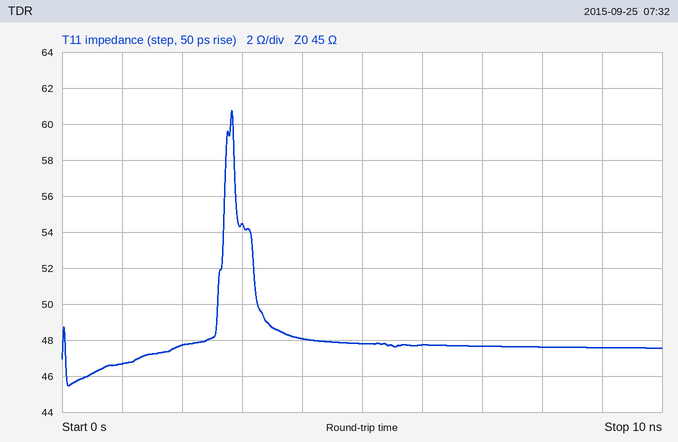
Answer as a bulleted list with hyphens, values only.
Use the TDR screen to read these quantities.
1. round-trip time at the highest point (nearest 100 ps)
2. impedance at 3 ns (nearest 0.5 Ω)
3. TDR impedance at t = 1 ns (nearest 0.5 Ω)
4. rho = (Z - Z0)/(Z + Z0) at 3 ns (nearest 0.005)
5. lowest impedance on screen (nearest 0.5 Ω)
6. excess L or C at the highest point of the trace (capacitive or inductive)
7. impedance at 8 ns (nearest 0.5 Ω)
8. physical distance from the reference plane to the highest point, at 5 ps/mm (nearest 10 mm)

- 2.8 ns
- 54.5 Ω
- 46.5 Ω
- +0.095
- 45.5 Ω
- inductive
- 47.5 Ω
- 280 mm
